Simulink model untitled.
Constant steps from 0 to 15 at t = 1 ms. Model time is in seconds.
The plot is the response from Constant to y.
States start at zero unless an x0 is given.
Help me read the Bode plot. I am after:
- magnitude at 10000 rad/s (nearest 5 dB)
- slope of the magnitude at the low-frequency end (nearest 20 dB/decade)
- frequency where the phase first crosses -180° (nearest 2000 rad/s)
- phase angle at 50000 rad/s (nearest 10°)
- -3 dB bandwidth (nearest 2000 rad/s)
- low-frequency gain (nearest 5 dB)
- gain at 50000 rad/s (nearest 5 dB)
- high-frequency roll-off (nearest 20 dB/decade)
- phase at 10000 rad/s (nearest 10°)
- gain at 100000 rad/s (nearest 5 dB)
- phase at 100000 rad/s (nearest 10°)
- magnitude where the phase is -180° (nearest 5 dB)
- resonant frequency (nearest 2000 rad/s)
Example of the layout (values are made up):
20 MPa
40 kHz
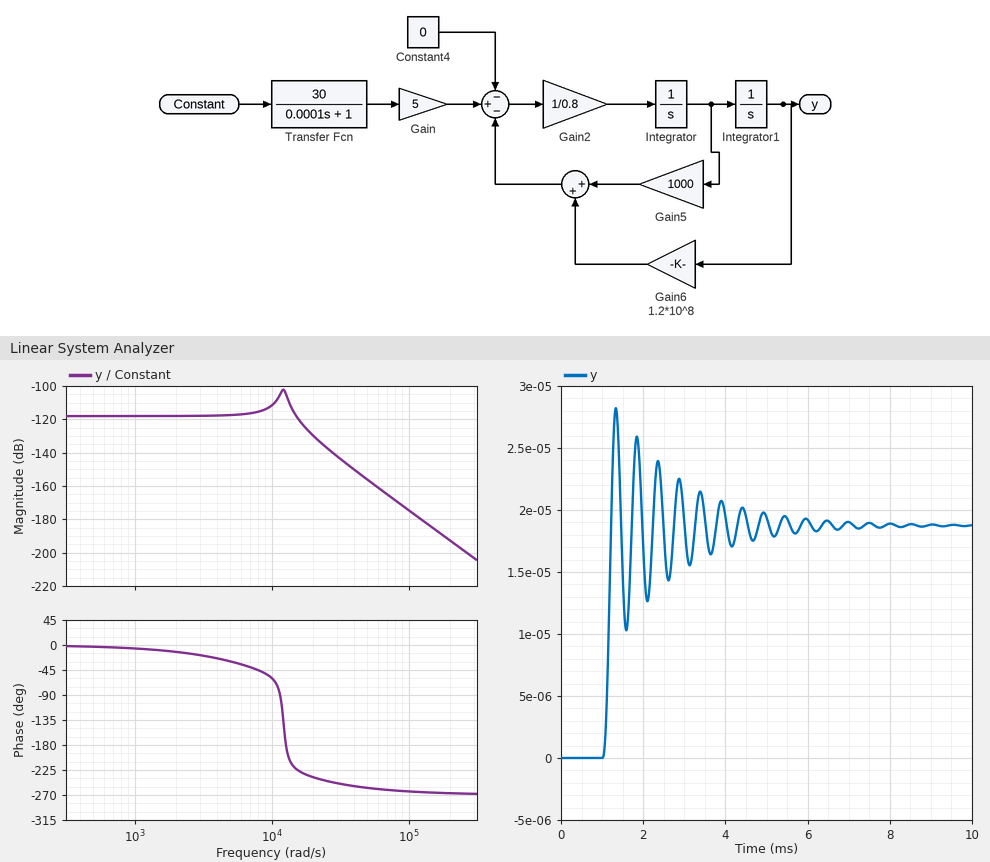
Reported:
-110 dB
0 dB/decade
12000 rad/s
-260°
16000 rad/s
-120 dB
-155 dB
-60 dB/decade
-60°
-175 dB
-260°
-105 dB
12000 rad/s
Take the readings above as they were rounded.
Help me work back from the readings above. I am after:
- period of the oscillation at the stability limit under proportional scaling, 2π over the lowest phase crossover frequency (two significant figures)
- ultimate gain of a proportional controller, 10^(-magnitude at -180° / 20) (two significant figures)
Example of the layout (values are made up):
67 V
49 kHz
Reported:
0.00052 s
180000
